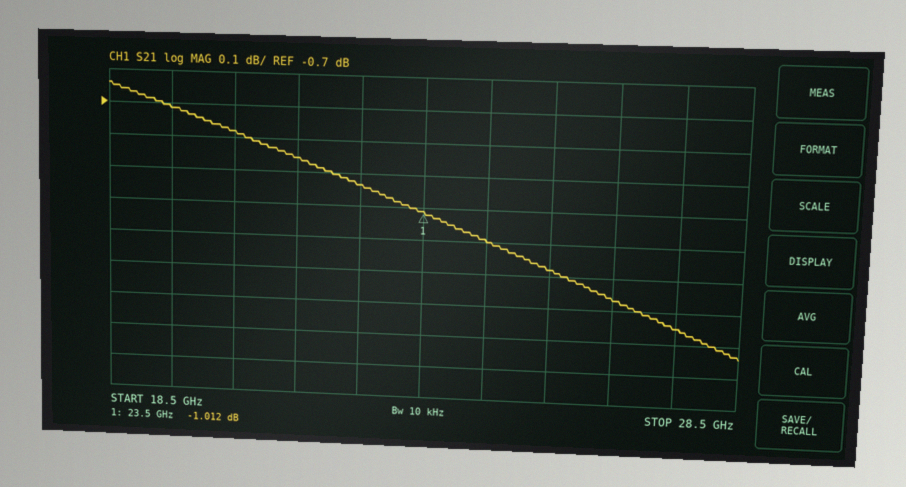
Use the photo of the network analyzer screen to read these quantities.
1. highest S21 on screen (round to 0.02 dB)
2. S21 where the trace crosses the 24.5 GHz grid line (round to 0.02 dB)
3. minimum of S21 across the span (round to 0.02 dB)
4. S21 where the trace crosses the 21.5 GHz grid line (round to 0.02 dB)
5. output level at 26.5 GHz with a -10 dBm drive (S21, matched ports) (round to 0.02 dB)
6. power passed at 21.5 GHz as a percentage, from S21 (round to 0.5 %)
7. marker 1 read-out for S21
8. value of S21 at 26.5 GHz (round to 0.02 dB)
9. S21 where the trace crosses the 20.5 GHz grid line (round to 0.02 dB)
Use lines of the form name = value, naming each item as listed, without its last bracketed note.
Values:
highest S21 on screen = -0.64 dB
S21 where the trace crosses the 24.5 GHz grid line = -1.10 dB
minimum of S21 across the span = -1.44 dB
S21 where the trace crosses the 21.5 GHz grid line = -0.86 dB
output level at 26.5 GHz with a -10 dBm drive (S21, matched ports) = -11.26 dBm
power passed at 21.5 GHz as a percentage, from S21 = 82.0 %
marker 1 read-out for S21 = -1.012 dB
value of S21 at 26.5 GHz = -1.26 dB
S21 where the trace crosses the 20.5 GHz grid line = -0.78 dB
